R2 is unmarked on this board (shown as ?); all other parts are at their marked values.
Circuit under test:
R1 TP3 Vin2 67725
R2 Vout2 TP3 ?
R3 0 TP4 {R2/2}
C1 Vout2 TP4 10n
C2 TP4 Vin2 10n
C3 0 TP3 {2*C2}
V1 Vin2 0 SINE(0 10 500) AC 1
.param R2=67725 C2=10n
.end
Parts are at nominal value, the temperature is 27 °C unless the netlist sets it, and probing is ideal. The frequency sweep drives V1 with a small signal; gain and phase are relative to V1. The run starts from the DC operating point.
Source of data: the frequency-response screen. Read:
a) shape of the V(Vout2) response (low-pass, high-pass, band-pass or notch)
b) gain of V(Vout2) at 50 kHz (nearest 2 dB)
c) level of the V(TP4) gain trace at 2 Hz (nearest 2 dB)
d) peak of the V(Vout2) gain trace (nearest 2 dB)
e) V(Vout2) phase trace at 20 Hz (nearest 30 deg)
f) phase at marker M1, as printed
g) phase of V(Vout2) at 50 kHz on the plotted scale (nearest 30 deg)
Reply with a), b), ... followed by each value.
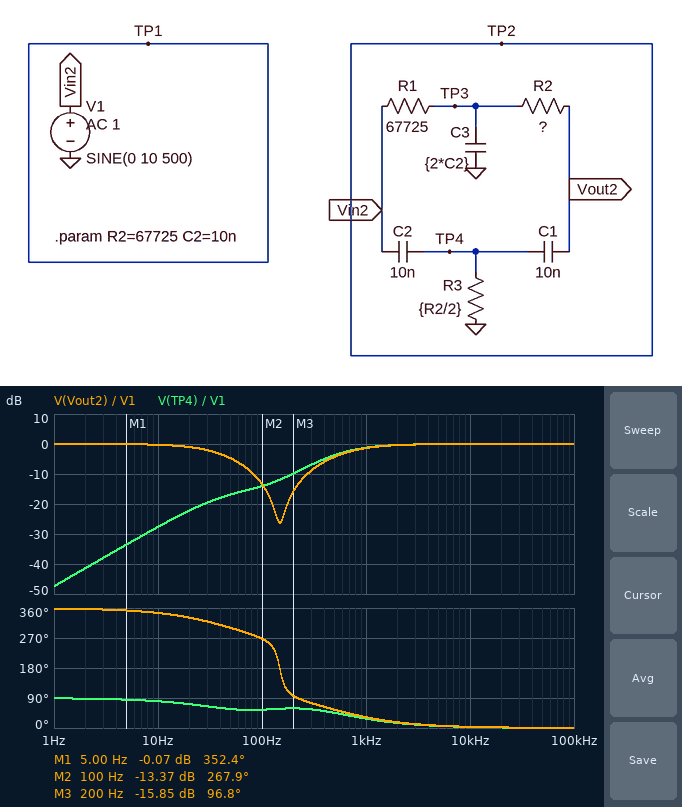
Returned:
a) notch
b) 0 dB
c) -42 dB
d) 0 dB
e) 330 deg
f) 352.4 deg
g) 0 deg
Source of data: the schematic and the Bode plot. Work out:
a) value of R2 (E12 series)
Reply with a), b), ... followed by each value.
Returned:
a) 220 kΩ
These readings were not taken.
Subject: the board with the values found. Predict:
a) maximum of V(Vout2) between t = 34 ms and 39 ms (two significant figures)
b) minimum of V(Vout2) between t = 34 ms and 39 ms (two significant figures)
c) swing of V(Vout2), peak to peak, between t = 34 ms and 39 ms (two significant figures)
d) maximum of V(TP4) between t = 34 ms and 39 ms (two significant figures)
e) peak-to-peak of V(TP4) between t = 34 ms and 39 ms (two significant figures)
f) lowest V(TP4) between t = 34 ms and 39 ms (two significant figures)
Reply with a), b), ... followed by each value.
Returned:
a) 6.1 V
b) -6.1 V
c) 12 V
d) 6.5 V
e) 13 V
f) -6.5 V
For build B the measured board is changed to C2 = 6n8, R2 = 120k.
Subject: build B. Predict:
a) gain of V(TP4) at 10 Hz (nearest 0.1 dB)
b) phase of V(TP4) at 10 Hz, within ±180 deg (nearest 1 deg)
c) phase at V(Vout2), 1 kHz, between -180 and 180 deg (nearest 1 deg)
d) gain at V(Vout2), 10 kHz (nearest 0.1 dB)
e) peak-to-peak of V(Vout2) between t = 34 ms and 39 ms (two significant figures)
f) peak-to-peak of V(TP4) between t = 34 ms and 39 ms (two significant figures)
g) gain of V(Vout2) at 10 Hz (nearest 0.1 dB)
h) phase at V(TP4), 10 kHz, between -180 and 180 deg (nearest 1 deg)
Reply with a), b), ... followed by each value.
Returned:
a) -29.1 dB
b) 81 deg
c) 48 deg
d) 0 dB
e) 7.7 V
f) 9.1 V
g) -0.2 dB
h) 5 deg
